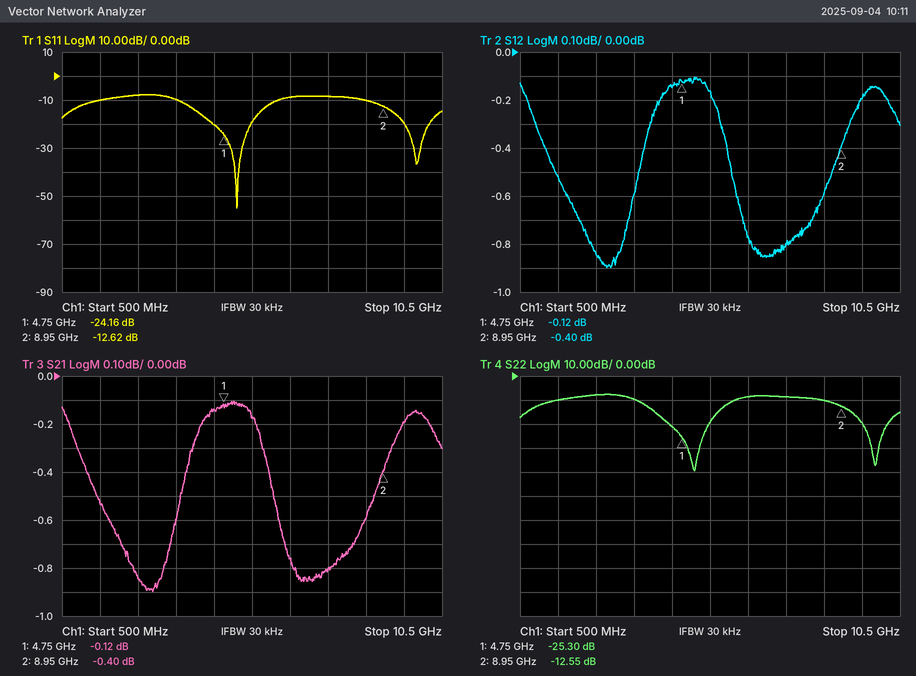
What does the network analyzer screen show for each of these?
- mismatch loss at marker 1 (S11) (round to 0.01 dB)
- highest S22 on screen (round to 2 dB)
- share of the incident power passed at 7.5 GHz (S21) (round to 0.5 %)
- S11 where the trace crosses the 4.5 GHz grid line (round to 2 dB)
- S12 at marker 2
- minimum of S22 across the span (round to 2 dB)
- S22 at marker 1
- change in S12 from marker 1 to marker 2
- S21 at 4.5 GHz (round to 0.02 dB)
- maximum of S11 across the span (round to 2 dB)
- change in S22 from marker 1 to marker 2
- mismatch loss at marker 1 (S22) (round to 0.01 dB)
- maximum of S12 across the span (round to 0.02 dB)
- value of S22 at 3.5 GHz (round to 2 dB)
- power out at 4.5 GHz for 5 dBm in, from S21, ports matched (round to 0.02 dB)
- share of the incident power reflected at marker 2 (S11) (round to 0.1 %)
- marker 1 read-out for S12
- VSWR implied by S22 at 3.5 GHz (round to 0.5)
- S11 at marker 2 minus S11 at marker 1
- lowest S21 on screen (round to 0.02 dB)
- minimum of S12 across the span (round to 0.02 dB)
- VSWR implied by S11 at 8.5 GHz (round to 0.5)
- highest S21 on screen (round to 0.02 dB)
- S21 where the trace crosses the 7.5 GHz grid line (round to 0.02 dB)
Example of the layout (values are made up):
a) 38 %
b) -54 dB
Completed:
a) 0.02 dB
b) -8 dB
c) 83.0 %
d) -20 dB
e) -0.40 dB
f) -40 dB
g) -25.30 dB
h) -0.28 dB
i) -0.14 dB
j) -8 dB
k) 12.75 dB
l) 0.01 dB
m) -0.10 dB
n) -10 dB
o) 4.86 dBm
p) 5.5 %
q) -0.12 dB
r) 2.0
s) 11.54 dB
t) -0.90 dB
u) -0.90 dB
v) 2.0
w) -0.10 dB
x) -0.80 dB
